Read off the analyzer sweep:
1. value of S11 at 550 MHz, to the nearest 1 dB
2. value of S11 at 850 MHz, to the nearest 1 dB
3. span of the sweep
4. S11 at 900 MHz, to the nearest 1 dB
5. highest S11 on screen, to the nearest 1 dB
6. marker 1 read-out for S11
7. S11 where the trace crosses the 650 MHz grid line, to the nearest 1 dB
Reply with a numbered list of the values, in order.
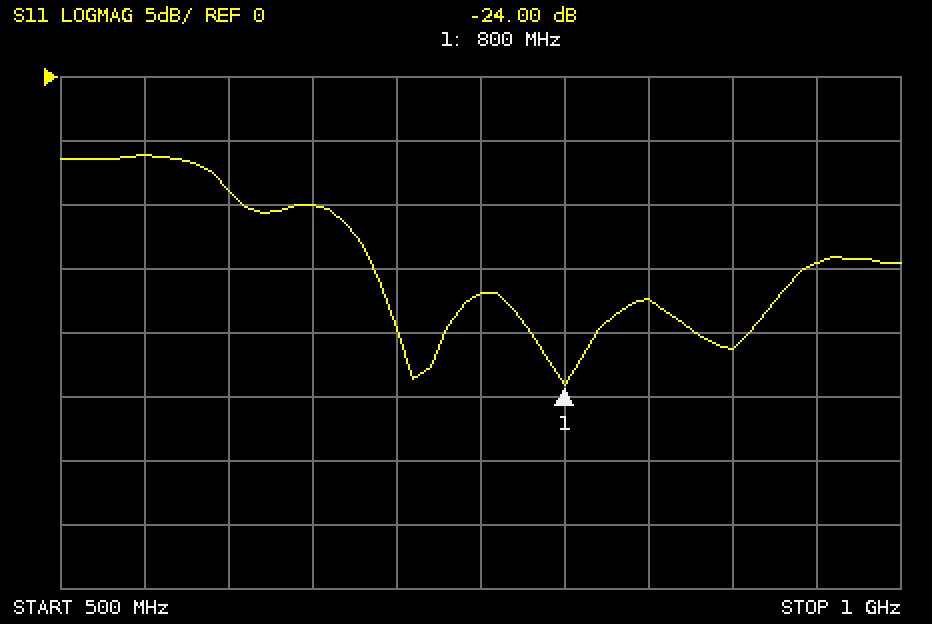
1. -6 dB
2. -17 dB
3. 500 MHz
4. -21 dB
5. -6 dB
6. -24.00 dB
7. -10 dB
